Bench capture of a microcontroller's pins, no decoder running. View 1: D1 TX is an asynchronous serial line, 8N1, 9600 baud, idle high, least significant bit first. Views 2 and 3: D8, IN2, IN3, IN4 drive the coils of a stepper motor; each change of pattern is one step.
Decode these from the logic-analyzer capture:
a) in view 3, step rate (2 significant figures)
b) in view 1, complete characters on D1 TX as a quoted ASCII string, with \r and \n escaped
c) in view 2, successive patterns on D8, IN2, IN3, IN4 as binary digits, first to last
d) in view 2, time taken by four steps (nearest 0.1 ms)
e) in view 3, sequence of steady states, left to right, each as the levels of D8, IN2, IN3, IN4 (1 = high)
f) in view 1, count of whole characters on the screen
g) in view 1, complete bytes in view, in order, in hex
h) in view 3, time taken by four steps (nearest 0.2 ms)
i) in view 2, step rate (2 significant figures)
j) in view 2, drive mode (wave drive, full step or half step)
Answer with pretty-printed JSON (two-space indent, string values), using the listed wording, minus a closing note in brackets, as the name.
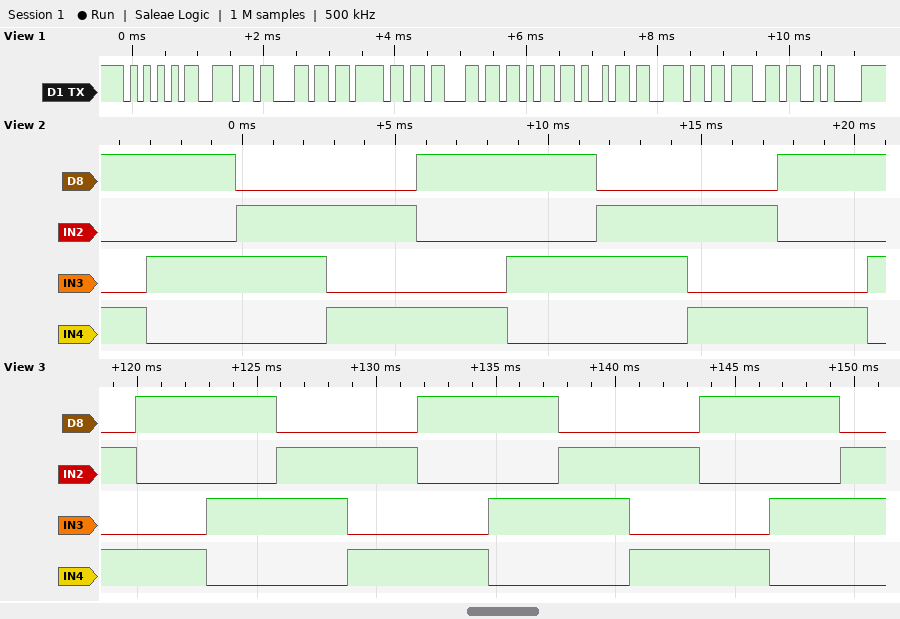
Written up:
{
  "in view 3, step rate": "340 steps/s",
  "in view 1, complete characters on D1 TX as a quoted ASCII string, with \\r and \\n escaped": "\"Unlocking\\n\"",
  "in view 2, successive patterns on D8, IN2, IN3, IN4 as binary digits, first to last": "1001 1010 0110 0101 1001 1010 0110 0101 1001 1010",
  "in view 2, time taken by four steps": "11.8 ms",
  "in view 3, sequence of steady states, left to right, each as the levels of D8, IN2, IN3, IN4": "0101 1001 1010 0110 0101 1001 1010 0110 0101 1001 1010 0110",
  "in view 1, count of whole characters on the screen": "10",
  "in view 1, complete bytes in view, in order, in hex": "55 6E 6C 6F 63 6B 69 6E 67 0A",
  "in view 3, time taken by four steps": "11.8 ms",
  "in view 2, step rate": "340 steps/s",
  "in view 2, drive mode": "full step"
}
